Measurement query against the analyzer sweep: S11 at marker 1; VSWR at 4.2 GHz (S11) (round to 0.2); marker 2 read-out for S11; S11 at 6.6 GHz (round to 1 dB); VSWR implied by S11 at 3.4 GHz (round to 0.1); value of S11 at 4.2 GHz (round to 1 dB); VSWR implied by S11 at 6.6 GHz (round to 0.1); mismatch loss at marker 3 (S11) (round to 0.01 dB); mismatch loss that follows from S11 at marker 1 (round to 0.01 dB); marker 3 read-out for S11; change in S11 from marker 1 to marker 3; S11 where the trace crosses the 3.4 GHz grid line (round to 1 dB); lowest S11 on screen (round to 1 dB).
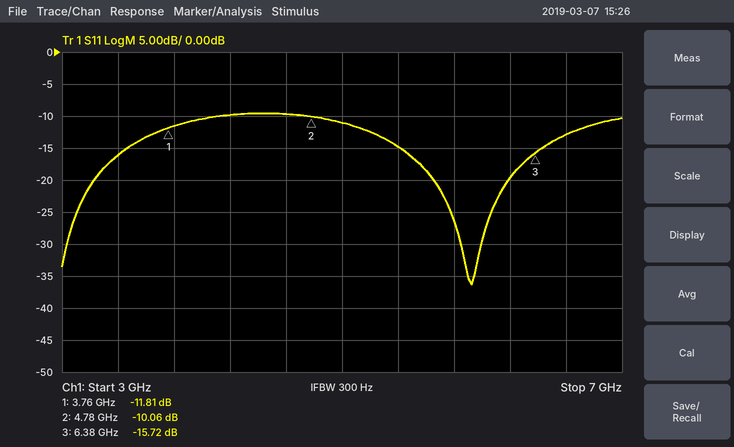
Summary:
-11.81 dB
2.0
-10.06 dB
-13 dB
1.4
-10 dB
1.6
0.12 dB
0.30 dB
-15.72 dB
-3.91 dB
-16 dB
-36 dB
